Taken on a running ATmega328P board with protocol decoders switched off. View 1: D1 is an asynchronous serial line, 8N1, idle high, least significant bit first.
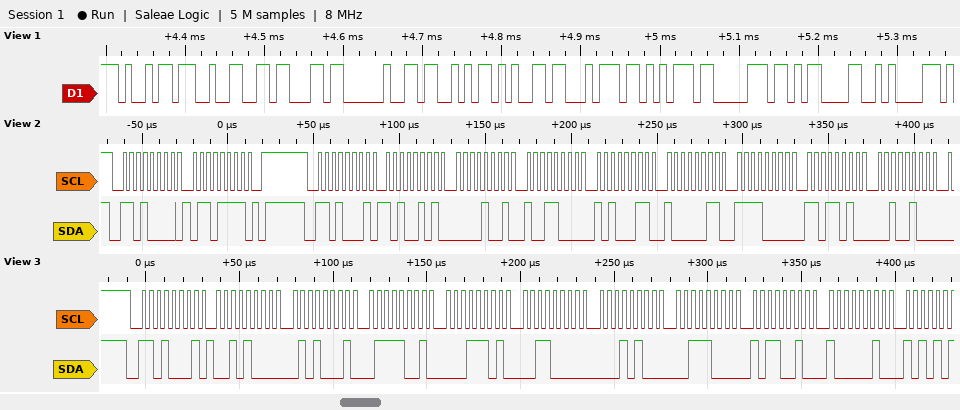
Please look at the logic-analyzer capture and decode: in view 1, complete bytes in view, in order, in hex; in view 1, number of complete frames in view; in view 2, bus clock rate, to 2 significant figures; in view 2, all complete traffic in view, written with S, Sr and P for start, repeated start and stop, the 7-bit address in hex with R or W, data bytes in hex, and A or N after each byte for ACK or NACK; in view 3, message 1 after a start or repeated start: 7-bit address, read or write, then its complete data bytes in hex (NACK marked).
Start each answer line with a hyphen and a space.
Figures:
- 69 32 63 20 53 65 74 75 70 0D 0A
- 11
- 250 kHz
- S 68W A 6F A P S 68R A A5 A 09 A 98 A A3 A 83 A F0 A DA A 24 A
- 0x68 read: 28 51 79 1D 30 14 38 B2 82
